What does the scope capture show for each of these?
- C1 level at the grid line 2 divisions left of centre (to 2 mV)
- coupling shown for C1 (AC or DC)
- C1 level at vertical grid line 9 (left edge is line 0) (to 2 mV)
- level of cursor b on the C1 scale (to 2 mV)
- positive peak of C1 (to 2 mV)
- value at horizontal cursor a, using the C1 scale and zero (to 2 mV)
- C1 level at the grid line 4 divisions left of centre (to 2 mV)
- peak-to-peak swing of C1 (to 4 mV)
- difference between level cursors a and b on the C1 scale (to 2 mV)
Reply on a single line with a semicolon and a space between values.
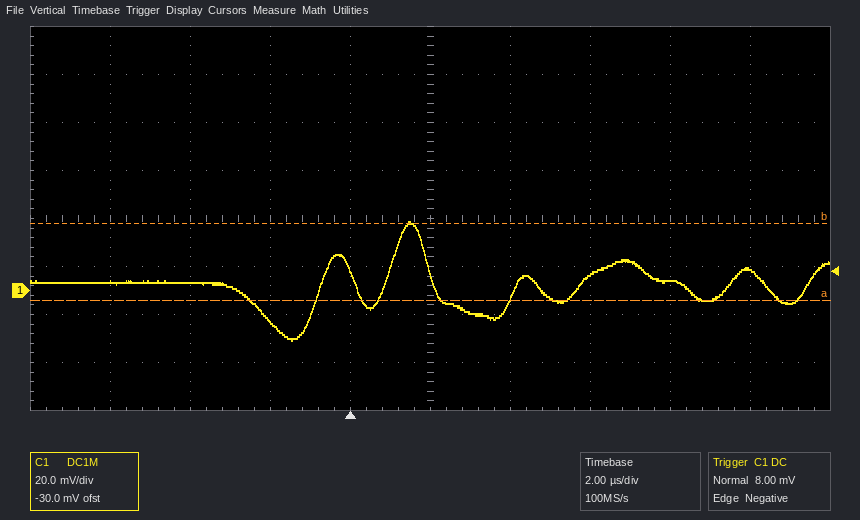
-12 mV; DC; 8 mV; 28 mV; 28 mV; -4 mV; 4 mV; 48 mV; 32 mV
